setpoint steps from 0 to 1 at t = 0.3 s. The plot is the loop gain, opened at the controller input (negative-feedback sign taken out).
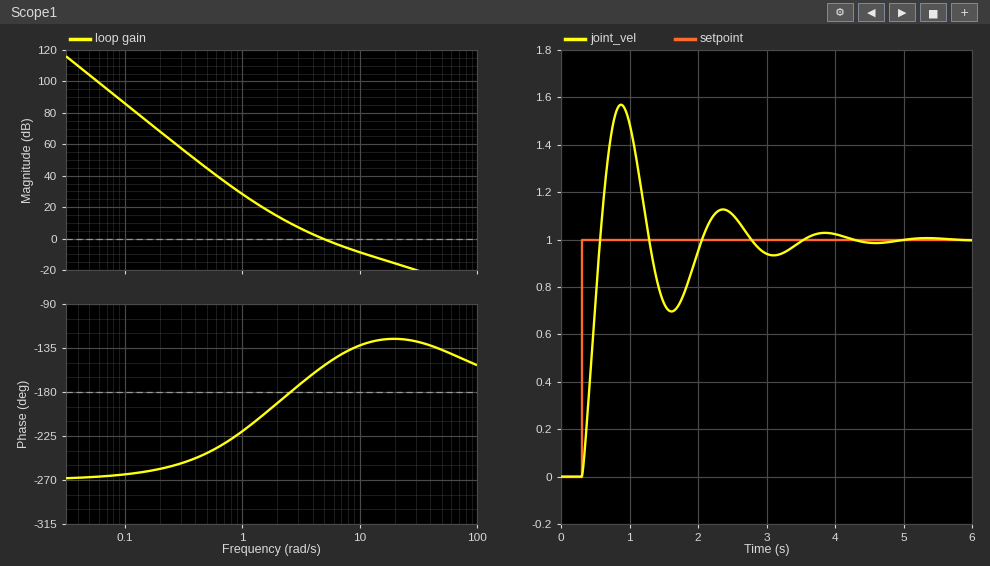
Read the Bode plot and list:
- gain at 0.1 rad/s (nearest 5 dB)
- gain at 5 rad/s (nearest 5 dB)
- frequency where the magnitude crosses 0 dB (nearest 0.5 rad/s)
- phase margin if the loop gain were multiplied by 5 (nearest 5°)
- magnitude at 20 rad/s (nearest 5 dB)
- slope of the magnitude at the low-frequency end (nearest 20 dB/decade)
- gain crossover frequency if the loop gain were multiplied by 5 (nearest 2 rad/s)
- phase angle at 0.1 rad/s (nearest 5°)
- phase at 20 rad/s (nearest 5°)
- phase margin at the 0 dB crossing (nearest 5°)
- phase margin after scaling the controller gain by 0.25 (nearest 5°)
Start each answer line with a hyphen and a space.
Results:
- 85 dB
- 0 dB
- 5.0 rad/s
- 55°
- -15 dB
- -60 dB/decade
- 16 rad/s
- -265°
- -125°
- 25°
- -5°
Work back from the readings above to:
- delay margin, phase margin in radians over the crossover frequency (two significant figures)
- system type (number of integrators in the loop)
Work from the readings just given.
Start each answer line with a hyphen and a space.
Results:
- 0.087 s
- 3
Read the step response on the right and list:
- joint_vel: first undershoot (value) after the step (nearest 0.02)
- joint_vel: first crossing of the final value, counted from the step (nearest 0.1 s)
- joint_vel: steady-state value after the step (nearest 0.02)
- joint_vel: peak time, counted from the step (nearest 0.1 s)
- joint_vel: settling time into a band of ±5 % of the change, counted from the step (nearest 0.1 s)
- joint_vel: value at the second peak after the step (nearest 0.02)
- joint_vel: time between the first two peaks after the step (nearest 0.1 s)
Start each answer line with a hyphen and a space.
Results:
- 0.70
- 0.3 s
- 1.00
- 0.6 s
- 3.0 s
- 1.12
- 1.5 s
